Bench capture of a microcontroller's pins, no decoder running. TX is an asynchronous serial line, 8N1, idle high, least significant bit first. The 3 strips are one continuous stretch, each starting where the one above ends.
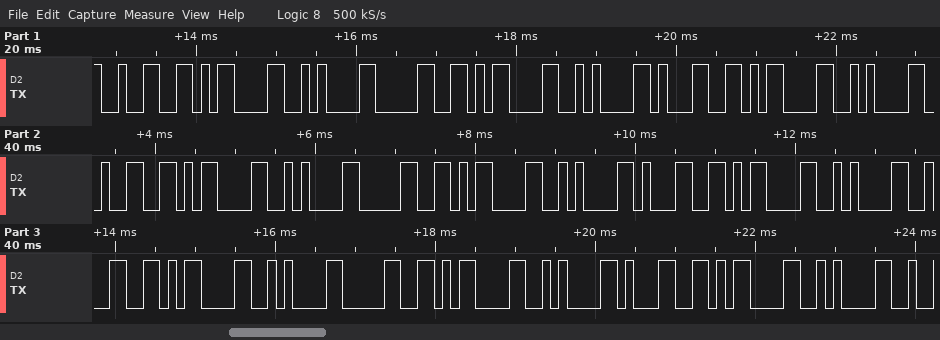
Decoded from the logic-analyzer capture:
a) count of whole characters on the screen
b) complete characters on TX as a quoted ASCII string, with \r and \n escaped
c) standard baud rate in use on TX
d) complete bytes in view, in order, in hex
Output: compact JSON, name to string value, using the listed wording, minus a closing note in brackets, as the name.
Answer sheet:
{"count of whole characters on the screen": "27", "complete characters on TX as a quoted ASCII string, with \\r and \\n escaped": "\"2\\r\\n0\\r\\n1\\r\\n2\\r\\n0\\r\\n1\\r\\n2\\r\\n0\\r\\n1\\r\\n\"", "standard baud rate in use on TX": "9600 baud", "complete bytes in view, in order, in hex": "32 0D 0A 30 0D 0A 31 0D 0A 32 0D 0A 30 0D 0A 31 0D 0A 32 0D 0A 30 0D 0A 31 0D 0A"}
